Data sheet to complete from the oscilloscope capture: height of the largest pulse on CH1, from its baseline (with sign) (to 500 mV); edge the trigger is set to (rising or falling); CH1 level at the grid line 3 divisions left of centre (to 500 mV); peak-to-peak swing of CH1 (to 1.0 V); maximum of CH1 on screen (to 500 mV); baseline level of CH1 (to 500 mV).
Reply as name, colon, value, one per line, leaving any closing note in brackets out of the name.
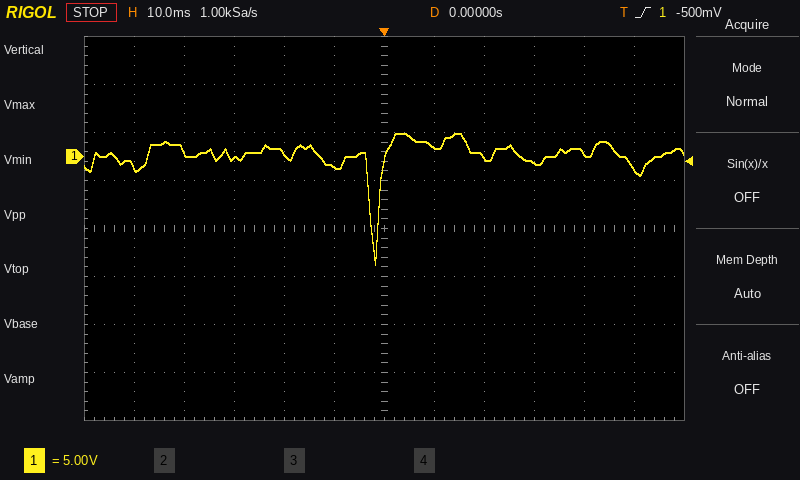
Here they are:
height of the largest pulse on CH1, from its baseline (with sign): -11.5 V
edge the trigger is set to: rising
CH1 level at the grid line 3 divisions left of centre: 0.0 V
peak-to-peak swing of CH1: 14.0 V
maximum of CH1 on screen: 2.5 V
baseline level of CH1: 500 mV
